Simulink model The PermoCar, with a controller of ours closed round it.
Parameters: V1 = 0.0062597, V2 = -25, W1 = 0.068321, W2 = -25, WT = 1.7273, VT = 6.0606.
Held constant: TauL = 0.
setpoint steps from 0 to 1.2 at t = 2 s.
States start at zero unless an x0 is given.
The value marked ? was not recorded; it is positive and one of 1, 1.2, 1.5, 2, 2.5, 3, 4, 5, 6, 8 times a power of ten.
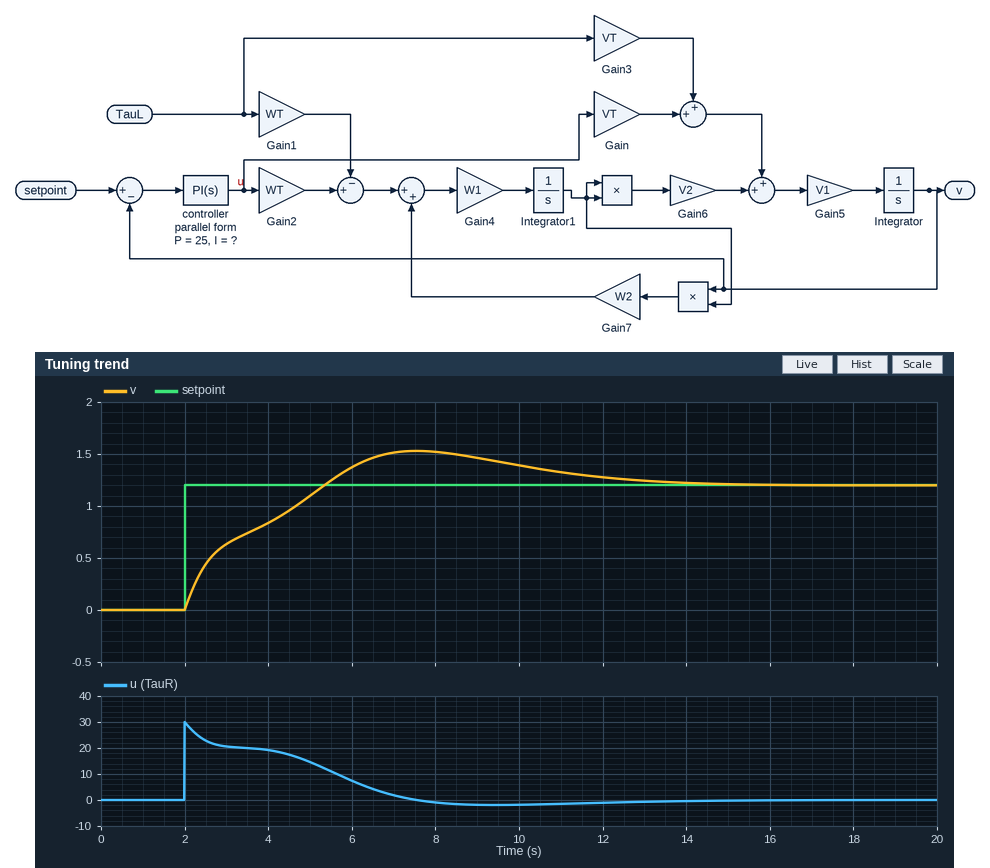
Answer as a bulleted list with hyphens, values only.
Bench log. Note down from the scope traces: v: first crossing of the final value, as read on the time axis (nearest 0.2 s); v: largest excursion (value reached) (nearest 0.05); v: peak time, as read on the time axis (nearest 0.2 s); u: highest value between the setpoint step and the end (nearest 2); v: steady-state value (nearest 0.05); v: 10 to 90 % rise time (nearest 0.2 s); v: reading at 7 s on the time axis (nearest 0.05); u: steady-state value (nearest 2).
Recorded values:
- 5.4 s
- 1.55
- 7.6 s
- 30
- 1.20
- 2.8 s
- 1.50
- 0
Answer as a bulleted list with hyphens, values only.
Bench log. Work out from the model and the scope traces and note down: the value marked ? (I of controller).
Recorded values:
- 8
